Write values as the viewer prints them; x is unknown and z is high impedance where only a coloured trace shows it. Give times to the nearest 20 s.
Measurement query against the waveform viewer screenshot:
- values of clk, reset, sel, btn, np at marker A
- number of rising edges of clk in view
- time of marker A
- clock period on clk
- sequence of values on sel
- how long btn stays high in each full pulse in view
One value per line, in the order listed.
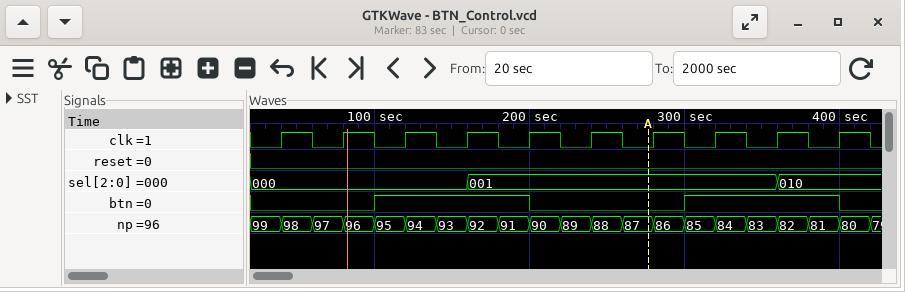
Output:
clk=0, reset=0, sel=001, btn=0, np=87
10
280 s
40 s
000, 001, 010
100 s, 100 s
